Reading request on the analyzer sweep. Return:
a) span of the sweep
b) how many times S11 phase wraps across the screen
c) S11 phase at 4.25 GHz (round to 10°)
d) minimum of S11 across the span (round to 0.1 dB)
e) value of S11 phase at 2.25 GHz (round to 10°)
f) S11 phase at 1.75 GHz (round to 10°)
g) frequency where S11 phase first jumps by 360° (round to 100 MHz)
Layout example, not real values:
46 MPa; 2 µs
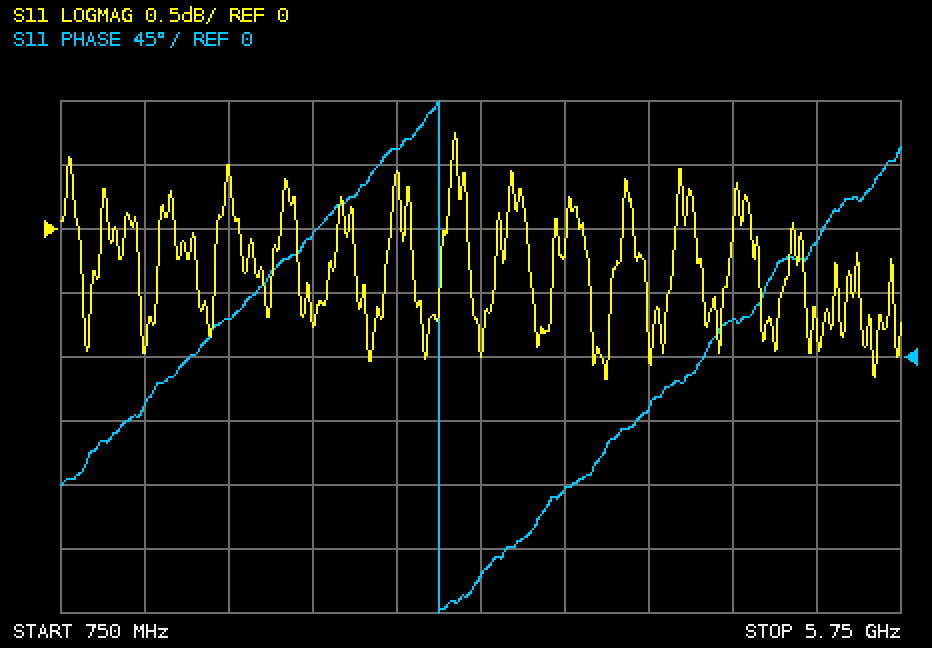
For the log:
5 GHz; 1; -40°; -1.2 dB; 90°; 30°; 3.0 GHz
